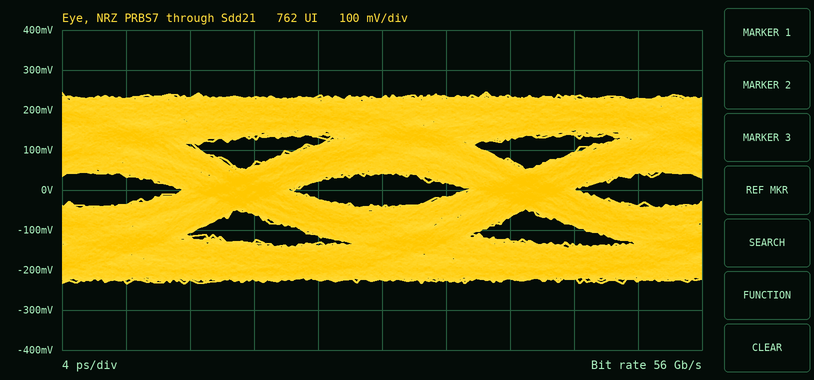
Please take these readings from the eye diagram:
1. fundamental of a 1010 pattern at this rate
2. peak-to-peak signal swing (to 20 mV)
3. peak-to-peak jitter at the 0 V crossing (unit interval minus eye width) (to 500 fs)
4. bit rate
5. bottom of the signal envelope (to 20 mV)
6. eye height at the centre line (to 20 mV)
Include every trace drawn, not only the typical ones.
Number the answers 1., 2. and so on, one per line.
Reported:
1. 28 GHz
2. 480 mV
3. 7.0 ps
4. 56 Gb/s
5. -240 mV
6. 80 mV
